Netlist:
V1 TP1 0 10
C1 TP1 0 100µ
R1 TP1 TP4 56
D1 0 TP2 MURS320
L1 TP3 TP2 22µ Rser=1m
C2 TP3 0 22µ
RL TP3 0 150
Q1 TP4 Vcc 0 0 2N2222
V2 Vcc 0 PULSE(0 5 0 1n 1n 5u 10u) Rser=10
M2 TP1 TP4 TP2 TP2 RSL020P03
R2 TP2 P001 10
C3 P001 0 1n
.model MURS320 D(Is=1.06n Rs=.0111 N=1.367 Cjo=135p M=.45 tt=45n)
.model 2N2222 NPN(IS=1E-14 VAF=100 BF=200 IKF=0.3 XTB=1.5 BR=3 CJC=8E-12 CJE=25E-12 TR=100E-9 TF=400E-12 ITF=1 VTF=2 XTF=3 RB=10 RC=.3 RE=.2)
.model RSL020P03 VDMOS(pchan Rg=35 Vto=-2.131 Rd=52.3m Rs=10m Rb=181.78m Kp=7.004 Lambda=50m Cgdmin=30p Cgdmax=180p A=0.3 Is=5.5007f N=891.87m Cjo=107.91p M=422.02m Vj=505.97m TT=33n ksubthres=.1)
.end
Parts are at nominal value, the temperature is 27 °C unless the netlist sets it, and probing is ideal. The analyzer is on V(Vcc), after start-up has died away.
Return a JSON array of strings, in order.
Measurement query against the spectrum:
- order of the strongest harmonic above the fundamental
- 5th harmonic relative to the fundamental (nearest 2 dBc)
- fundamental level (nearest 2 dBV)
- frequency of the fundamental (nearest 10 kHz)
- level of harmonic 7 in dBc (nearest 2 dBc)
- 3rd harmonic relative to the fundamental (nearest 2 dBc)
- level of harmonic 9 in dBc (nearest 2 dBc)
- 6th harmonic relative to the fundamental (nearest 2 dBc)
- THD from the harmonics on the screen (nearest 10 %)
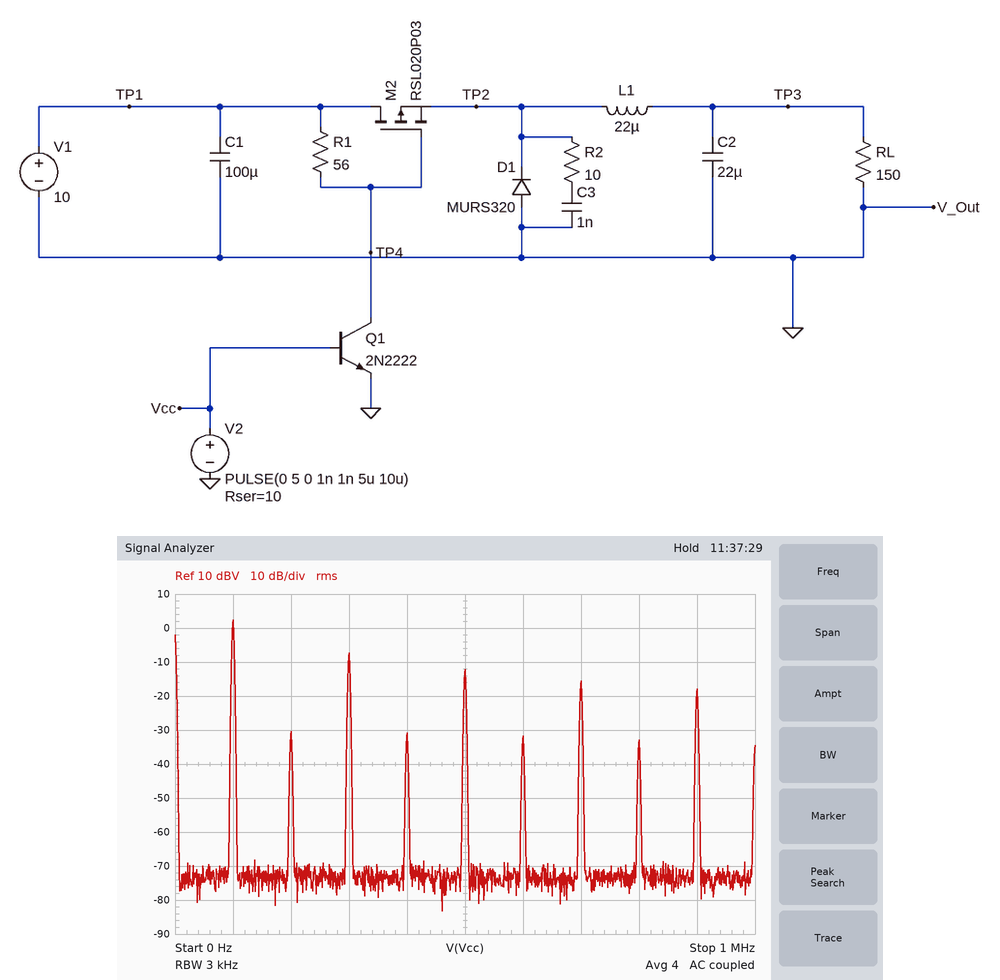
["3", "-14 dBc", "2 dBV", "100 kHz", "-18 dBc", "-10 dBc", "-20 dBc", "-34 dBc", "40 %"]
